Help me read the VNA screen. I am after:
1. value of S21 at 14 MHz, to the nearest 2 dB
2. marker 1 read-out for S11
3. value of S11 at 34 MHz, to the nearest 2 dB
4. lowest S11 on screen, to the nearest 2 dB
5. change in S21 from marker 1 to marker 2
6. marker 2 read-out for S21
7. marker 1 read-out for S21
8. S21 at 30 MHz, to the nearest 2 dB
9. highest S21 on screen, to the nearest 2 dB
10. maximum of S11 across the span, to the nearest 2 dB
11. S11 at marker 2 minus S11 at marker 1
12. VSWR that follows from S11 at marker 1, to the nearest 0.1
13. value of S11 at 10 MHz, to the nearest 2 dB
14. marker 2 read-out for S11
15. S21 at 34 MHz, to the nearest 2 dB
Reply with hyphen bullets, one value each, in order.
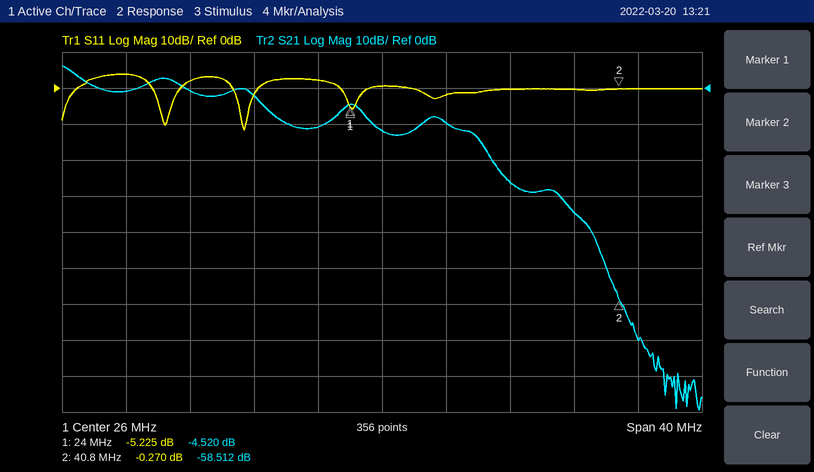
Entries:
- 0 dB
- -5.225 dB
- 0 dB
- -12 dB
- -53.992 dB
- -58.512 dB
- -4.520 dB
- -10 dB
- 6 dB
- 4 dB
- 4.955 dB
- 3.4
- 4 dB
- -0.270 dB
- -26 dB
